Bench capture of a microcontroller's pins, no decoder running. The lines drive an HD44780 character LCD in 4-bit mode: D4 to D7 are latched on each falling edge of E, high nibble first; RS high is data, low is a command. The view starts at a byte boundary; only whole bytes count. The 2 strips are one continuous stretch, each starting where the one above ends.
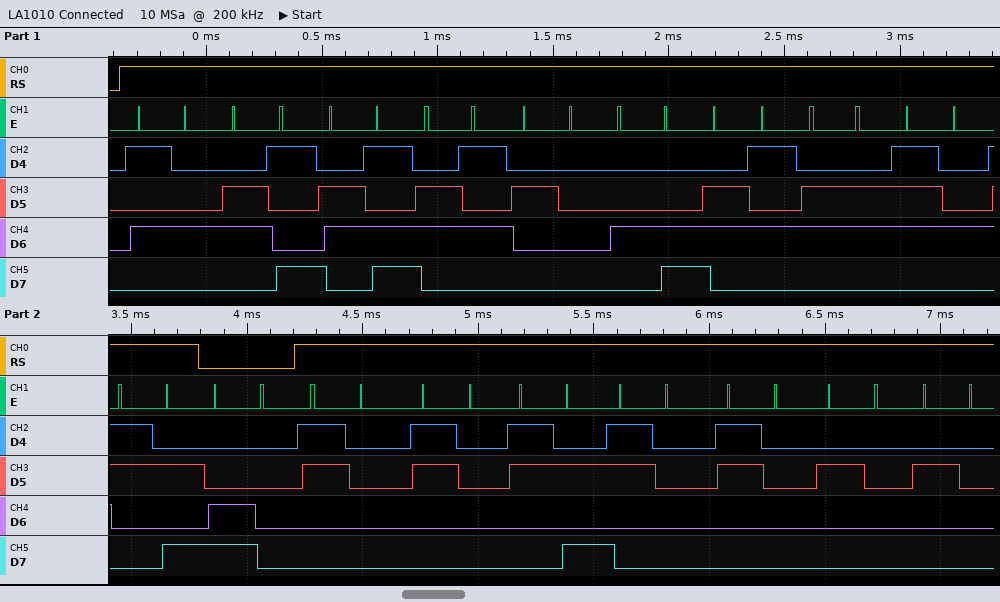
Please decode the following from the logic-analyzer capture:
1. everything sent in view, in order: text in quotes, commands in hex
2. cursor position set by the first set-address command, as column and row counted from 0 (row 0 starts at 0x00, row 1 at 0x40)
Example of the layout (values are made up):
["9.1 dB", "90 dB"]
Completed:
["\"Time Left:\" 0xC0 \"00:00  \"", "column 0, row 1"]
